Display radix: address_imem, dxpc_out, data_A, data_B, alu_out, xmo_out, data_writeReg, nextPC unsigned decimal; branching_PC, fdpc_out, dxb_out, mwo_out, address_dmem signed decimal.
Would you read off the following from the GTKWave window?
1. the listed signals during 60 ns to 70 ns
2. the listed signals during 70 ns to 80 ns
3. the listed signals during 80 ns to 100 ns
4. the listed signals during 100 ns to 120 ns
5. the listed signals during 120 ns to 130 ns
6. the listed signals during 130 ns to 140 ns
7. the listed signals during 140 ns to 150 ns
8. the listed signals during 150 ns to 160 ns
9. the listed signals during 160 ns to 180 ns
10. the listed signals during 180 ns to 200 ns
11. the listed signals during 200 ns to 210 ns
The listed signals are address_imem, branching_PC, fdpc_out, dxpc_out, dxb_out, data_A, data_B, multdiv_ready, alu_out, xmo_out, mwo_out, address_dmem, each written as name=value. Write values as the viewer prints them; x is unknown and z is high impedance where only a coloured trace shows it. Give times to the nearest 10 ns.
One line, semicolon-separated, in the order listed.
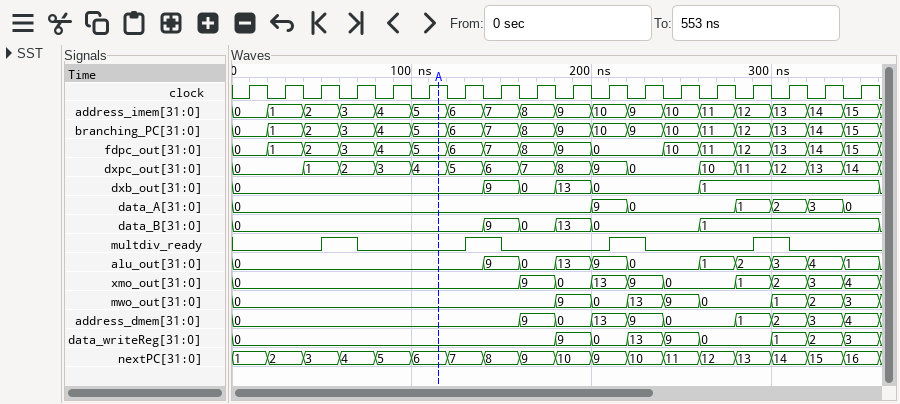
address_imem=3, branching_PC=3, fdpc_out=3, dxpc_out=2, dxb_out=0, data_A=0, data_B=0, multdiv_ready=1, alu_out=0, xmo_out=0, mwo_out=0, address_dmem=0; address_imem=3, branching_PC=3, fdpc_out=3, dxpc_out=2, dxb_out=0, data_A=0, data_B=0, multdiv_ready=0, alu_out=0, xmo_out=0, mwo_out=0, address_dmem=0; address_imem=4, branching_PC=4, fdpc_out=4, dxpc_out=3, dxb_out=0, data_A=0, data_B=0, multdiv_ready=0, alu_out=0, xmo_out=0, mwo_out=0, address_dmem=0; address_imem=5, branching_PC=5, fdpc_out=5, dxpc_out=4, dxb_out=0, data_A=0, data_B=0, multdiv_ready=0, alu_out=0, xmo_out=0, mwo_out=0, address_dmem=0; address_imem=6, branching_PC=6, fdpc_out=6, dxpc_out=5, dxb_out=0, data_A=0, data_B=0, multdiv_ready=0, alu_out=0, xmo_out=0, mwo_out=0, address_dmem=0; address_imem=6, branching_PC=6, fdpc_out=6, dxpc_out=5, dxb_out=0, data_A=0, data_B=0, multdiv_ready=1, alu_out=0, xmo_out=0, mwo_out=0, address_dmem=0; address_imem=7, branching_PC=7, fdpc_out=7, dxpc_out=6, dxb_out=9, data_A=0, data_B=9, multdiv_ready=1, alu_out=9, xmo_out=0, mwo_out=0, address_dmem=0; address_imem=7, branching_PC=7, fdpc_out=7, dxpc_out=6, dxb_out=9, data_A=0, data_B=9, multdiv_ready=0, alu_out=9, xmo_out=0, mwo_out=0, address_dmem=0; address_imem=8, branching_PC=8, fdpc_out=8, dxpc_out=7, dxb_out=0, data_A=0, data_B=0, multdiv_ready=0, alu_out=0, xmo_out=9, mwo_out=0, address_dmem=9; address_imem=9, branching_PC=9, fdpc_out=9, dxpc_out=8, dxb_out=13, data_A=0, data_B=13, multdiv_ready=0, alu_out=13, xmo_out=0, mwo_out=9, address_dmem=0; address_imem=10, branching_PC=10, fdpc_out=0, dxpc_out=9, dxb_out=0, data_A=9, data_B=0, multdiv_ready=0, alu_out=9, xmo_out=13, mwo_out=0, address_dmem=13
